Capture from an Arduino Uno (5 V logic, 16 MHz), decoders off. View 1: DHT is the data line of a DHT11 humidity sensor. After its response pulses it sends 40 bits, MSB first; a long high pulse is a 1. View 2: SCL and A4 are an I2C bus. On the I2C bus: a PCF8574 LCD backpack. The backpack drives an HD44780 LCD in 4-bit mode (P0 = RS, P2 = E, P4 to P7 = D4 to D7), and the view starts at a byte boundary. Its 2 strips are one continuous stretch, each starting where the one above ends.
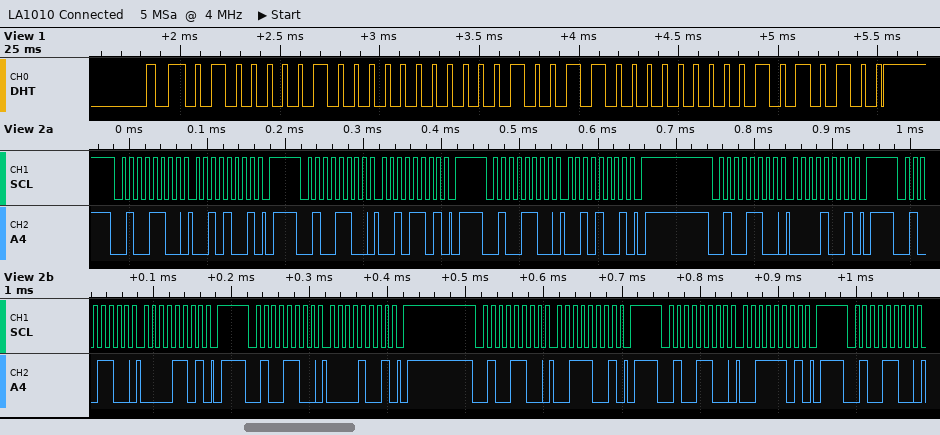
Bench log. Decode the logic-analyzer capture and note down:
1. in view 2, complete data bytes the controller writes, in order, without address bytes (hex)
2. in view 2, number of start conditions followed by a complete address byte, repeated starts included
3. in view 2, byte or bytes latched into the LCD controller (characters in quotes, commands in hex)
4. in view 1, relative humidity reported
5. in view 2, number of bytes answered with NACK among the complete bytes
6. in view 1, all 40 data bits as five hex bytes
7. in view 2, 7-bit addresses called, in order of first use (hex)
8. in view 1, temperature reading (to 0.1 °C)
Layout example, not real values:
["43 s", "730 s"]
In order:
["29 2D 29 09 0D 09 39 3D", "9", "' '", "65 %", "0", "41 00 13 00 54", "0x26", "19.0 °C"]
